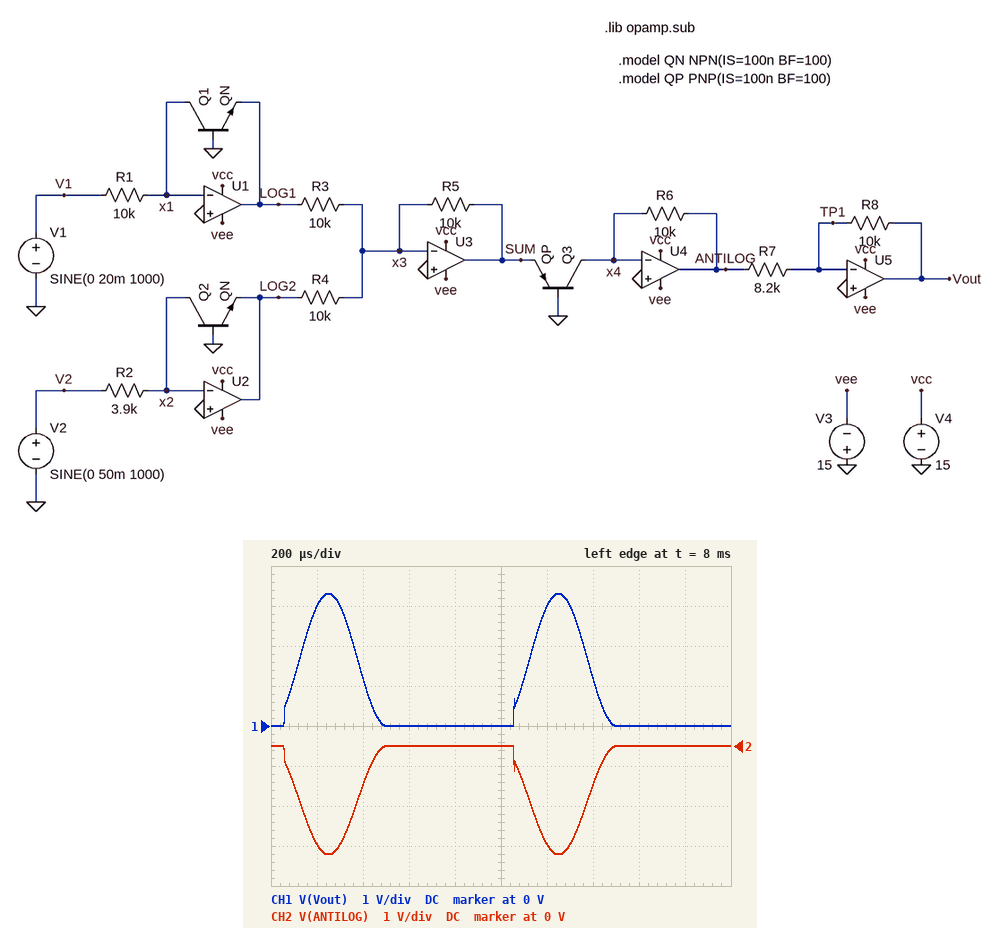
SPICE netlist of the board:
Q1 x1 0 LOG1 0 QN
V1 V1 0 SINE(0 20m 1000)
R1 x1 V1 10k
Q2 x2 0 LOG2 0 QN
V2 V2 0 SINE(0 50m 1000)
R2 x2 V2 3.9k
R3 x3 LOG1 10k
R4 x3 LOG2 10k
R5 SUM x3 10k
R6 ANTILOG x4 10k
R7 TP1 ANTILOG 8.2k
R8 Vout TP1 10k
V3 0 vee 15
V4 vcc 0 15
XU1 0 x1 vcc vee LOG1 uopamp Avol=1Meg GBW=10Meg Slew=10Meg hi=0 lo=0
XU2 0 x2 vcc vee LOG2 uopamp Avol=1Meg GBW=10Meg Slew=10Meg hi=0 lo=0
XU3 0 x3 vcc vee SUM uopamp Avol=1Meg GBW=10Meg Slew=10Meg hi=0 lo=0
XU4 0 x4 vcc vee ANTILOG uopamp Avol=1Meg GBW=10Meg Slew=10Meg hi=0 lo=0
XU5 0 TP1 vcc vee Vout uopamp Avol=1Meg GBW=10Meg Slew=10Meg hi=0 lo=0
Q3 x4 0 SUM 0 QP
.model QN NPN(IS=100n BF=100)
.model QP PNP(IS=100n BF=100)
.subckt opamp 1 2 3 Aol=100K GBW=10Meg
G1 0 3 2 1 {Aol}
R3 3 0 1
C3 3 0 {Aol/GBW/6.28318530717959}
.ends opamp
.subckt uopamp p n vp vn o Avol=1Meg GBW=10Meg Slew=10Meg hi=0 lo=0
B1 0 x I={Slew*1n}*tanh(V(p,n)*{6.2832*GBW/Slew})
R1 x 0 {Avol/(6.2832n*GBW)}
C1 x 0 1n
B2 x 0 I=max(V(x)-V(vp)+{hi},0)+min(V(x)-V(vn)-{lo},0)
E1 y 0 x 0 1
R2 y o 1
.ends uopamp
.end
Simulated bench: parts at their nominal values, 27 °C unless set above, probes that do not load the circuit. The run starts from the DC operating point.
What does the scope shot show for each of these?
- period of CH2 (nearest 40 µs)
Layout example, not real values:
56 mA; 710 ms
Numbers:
1.00 ms
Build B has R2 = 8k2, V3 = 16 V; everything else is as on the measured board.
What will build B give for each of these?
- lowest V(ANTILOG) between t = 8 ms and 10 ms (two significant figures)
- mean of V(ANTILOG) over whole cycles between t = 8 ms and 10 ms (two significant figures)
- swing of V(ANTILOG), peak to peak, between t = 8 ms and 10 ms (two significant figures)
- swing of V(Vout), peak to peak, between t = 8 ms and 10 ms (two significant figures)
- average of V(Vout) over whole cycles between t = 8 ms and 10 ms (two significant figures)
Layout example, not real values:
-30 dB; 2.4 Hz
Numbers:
-1.3 V; -330 mV; 1.3 V; 1.6 V; 400 mV
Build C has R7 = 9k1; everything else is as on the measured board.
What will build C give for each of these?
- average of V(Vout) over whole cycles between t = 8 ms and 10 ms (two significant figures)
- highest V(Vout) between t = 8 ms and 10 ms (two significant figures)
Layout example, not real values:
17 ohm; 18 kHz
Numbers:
750 mV; 3.0 V
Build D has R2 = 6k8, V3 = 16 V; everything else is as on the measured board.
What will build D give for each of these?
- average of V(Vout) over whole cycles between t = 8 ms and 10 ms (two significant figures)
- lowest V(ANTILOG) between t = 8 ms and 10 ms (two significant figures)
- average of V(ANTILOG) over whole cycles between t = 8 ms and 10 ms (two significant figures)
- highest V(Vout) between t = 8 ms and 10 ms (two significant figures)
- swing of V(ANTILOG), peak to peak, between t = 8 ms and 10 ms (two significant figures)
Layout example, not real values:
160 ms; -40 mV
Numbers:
480 mV; -1.6 V; -390 mV; 1.9 V; 1.6 V
